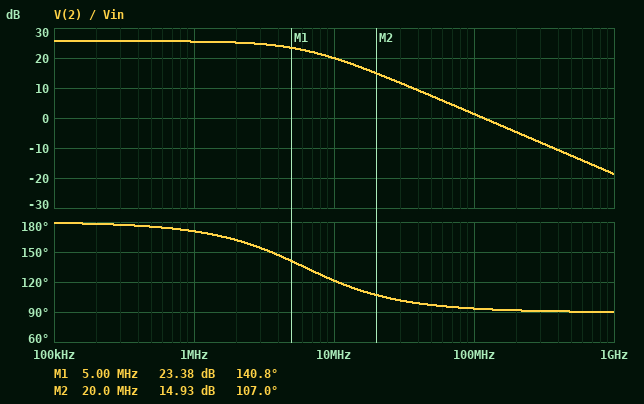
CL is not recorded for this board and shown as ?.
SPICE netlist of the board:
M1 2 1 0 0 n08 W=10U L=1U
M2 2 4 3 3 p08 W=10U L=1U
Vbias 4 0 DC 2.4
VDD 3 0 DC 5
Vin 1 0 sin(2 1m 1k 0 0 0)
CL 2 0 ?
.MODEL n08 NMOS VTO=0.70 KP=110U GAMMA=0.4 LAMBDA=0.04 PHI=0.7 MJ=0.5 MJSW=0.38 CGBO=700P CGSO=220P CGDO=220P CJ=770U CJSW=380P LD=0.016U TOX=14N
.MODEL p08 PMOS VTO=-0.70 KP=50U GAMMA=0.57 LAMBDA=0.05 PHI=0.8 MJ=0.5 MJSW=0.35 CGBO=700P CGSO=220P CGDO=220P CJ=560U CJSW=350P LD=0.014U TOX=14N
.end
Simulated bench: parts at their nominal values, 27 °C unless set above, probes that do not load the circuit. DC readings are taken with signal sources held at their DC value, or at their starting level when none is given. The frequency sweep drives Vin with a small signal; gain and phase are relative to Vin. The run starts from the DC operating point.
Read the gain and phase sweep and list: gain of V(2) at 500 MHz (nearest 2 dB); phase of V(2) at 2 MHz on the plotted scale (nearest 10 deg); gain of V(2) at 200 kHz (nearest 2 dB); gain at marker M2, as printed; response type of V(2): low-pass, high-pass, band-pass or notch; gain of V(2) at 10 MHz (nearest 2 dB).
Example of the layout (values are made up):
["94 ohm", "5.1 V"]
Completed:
["-12 dB", "160 deg", "26 dB", "14.93 dB", "low-pass", "20 dB"]
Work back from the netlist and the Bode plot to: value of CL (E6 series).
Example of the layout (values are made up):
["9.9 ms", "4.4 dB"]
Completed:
["2.2 pF"]
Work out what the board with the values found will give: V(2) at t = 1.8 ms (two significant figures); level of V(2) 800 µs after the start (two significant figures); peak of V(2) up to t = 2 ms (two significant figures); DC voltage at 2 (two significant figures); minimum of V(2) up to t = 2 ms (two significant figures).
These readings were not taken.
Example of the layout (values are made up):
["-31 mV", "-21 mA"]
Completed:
["2.4 V", "2.4 V", "2.4 V", "2.4 V", "2.3 V"]
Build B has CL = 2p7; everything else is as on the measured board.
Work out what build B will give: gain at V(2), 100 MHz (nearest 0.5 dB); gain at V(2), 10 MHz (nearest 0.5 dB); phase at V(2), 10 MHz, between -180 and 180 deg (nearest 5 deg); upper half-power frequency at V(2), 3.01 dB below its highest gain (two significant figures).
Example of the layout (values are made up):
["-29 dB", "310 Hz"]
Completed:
["-0.5 dB", "18.5 dB", "115 deg", "5.0 MHz"]
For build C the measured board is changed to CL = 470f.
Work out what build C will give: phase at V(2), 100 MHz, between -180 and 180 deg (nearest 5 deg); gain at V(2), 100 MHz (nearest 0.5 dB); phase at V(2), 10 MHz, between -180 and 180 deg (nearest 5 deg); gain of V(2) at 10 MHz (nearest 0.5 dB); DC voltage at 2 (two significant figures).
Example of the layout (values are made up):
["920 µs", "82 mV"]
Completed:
["105 deg", "14.5 dB", "160 deg", "25.0 dB", "2.4 V"]
